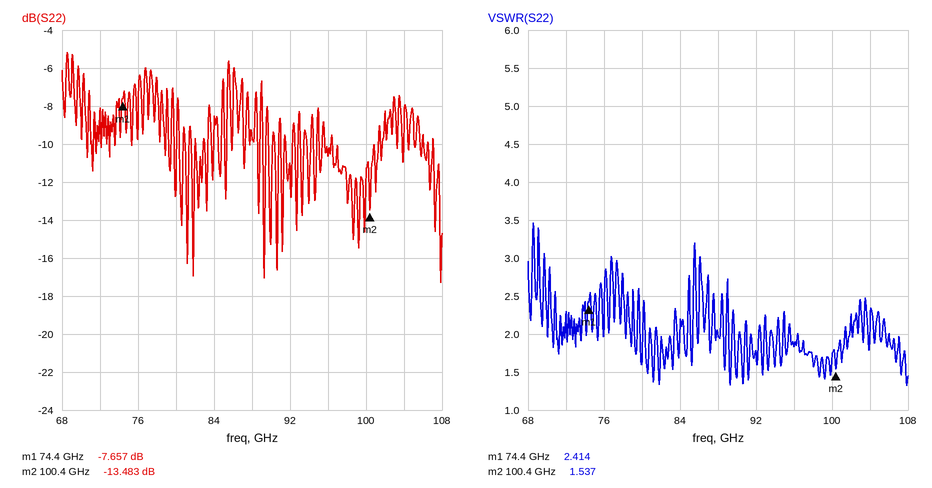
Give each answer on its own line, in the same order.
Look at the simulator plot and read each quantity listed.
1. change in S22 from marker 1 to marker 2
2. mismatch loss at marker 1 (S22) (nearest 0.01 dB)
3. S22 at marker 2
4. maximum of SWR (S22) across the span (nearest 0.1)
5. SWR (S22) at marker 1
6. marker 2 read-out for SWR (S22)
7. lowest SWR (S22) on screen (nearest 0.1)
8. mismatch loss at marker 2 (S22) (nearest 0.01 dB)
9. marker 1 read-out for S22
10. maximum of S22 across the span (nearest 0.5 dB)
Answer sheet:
-5.826 dB
0.82 dB
-13.483 dB
3.5
2.414
1.537
1.3
0.20 dB
-7.657 dB
-5.0 dB
